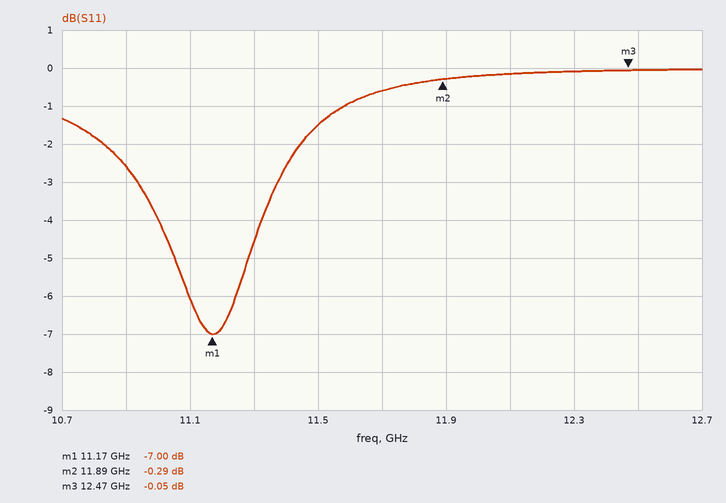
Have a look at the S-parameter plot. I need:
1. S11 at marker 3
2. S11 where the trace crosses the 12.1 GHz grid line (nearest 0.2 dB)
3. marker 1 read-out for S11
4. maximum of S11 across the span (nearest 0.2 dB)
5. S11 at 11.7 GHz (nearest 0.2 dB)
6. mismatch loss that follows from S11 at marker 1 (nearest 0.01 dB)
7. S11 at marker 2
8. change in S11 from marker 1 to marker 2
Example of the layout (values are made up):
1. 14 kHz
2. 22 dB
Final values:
1. -0.05 dB
2. -0.2 dB
3. -7.00 dB
4. 0.0 dB
5. -0.6 dB
6. 0.97 dB
7. -0.29 dB
8. 6.71 dB
